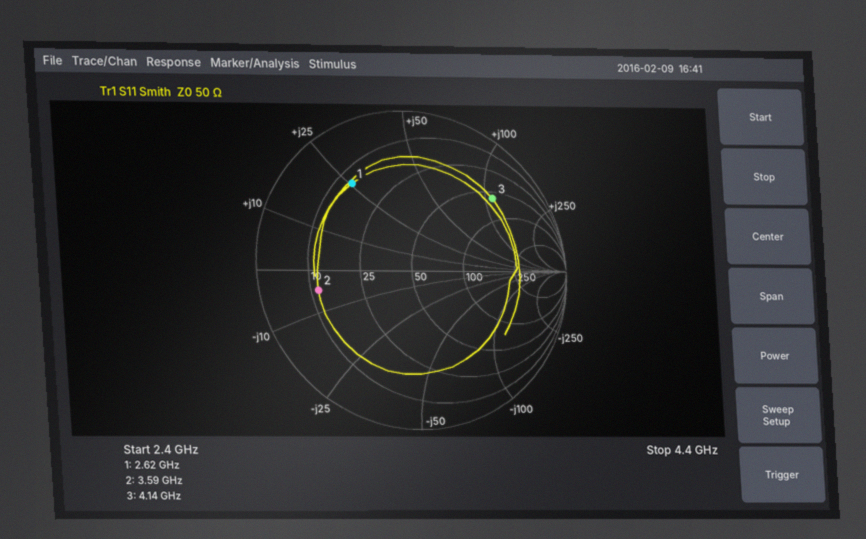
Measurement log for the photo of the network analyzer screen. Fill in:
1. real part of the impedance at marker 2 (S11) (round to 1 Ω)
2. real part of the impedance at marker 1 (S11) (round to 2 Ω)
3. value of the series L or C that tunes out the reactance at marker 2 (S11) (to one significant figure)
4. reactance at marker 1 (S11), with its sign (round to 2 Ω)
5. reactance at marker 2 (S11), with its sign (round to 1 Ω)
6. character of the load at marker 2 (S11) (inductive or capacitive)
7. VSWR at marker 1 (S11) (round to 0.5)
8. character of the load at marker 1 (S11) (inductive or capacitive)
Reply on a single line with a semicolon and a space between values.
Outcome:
12 Ω; 14 Ω; 200 pH; +26 Ω; -5 Ω; capacitive; 4.5; inductive
